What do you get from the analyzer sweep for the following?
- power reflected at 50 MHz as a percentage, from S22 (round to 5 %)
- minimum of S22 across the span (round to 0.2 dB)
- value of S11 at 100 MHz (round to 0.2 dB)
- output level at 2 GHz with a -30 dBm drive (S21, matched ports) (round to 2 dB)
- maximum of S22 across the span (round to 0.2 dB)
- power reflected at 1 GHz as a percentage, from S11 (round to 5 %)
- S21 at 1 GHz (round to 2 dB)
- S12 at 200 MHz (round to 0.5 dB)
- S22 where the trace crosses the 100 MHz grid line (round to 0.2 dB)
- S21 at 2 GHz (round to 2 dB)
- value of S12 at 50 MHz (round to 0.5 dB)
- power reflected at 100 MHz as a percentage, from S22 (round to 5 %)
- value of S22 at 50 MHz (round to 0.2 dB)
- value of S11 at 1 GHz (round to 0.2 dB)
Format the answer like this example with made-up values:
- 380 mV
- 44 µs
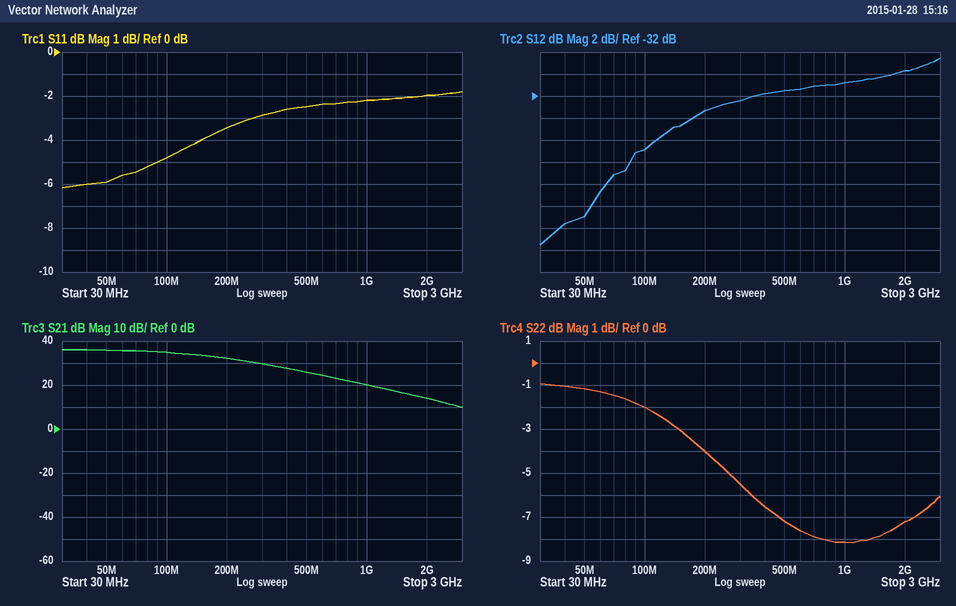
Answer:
- 75 %
- -8.2 dB
- -4.8 dB
- -16 dBm
- -1.0 dB
- 60 %
- 20 dB
- -33.5 dB
- -2.0 dB
- 14 dB
- -43.0 dB
- 65 %
- -1.2 dB
- -2.2 dB
